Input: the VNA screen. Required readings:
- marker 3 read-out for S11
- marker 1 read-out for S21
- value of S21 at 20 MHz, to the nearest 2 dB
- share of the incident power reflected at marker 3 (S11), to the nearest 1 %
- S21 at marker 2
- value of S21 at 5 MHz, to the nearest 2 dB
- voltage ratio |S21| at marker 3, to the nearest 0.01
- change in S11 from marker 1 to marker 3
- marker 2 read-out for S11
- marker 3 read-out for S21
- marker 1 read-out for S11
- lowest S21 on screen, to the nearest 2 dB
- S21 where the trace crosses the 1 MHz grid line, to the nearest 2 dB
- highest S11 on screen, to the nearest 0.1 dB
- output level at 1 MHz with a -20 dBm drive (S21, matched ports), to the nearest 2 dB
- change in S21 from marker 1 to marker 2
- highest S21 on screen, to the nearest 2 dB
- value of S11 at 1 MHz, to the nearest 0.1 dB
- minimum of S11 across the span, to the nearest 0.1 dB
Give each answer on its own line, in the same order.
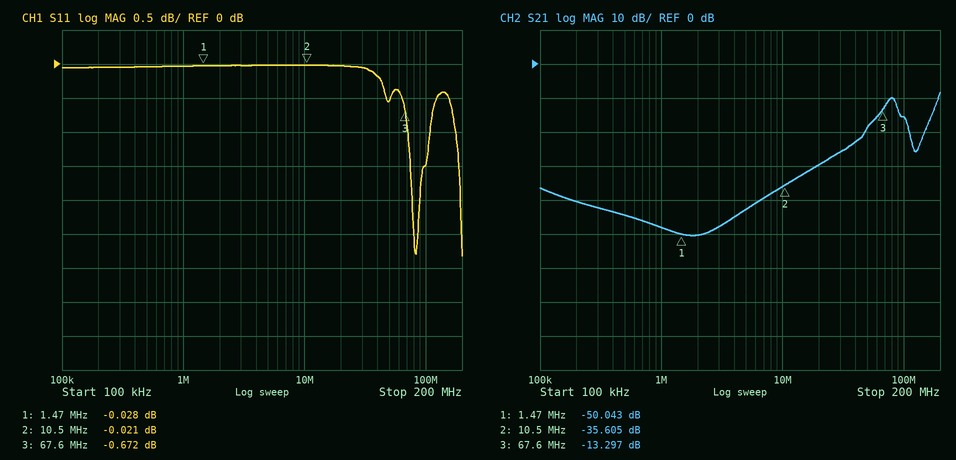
-0.672 dB
-50.043 dB
-30 dB
86 %
-35.605 dB
-42 dB
0.22
-0.644 dB
-0.021 dB
-13.297 dB
-0.028 dB
-50 dB
-48 dB
0.0 dB
-68 dBm
14.438 dB
-8 dB
0.0 dB
-2.8 dB
